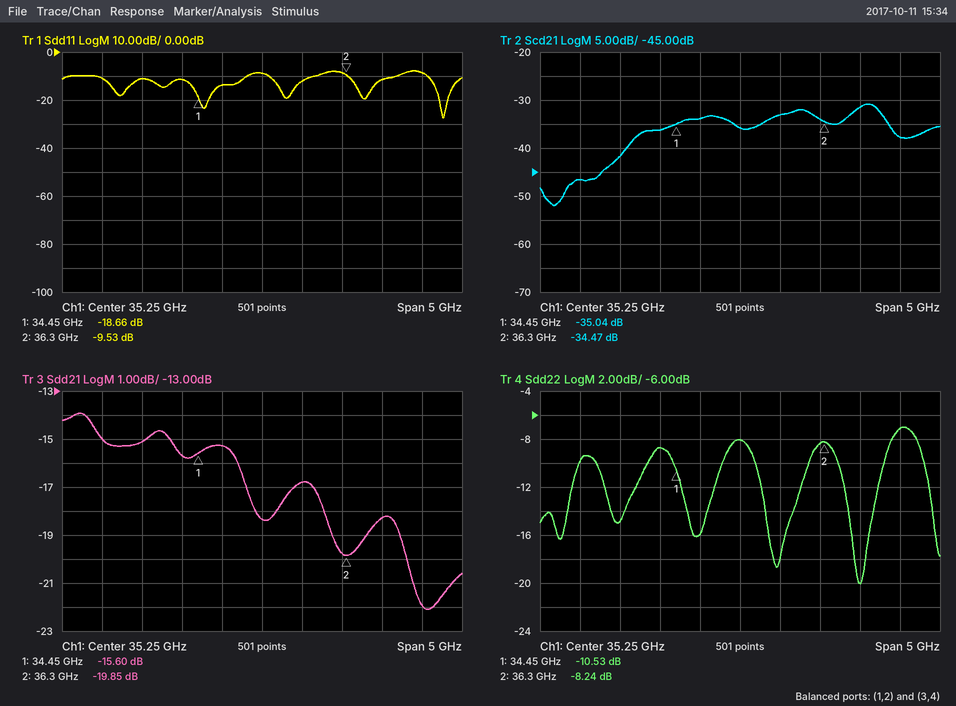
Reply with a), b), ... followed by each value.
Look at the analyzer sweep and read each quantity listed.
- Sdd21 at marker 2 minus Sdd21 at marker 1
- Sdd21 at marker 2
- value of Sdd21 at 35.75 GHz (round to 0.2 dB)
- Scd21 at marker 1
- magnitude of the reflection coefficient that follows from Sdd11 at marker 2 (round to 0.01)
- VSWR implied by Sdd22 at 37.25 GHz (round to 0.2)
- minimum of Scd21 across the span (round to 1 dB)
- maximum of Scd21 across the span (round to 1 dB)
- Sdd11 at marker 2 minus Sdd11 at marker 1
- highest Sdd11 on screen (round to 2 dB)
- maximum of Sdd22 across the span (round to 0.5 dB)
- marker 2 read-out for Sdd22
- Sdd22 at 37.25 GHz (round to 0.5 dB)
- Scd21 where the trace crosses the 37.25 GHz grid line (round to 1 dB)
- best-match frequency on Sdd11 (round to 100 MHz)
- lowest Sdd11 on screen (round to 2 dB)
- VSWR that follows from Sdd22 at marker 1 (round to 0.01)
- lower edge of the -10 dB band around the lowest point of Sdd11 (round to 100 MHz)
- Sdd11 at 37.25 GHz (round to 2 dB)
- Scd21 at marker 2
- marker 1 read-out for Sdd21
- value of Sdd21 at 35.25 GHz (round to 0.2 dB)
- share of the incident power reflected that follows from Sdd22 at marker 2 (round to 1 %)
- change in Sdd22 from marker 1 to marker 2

a) -4.25 dB
b) -19.85 dB
c) -16.8 dB
d) -35.04 dB
e) 0.33
f) 2.6
g) -52 dB
h) -31 dB
i) 9.13 dB
j) -8 dB
k) -7.0 dB
l) -8.24 dB
m) -7.0 dB
n) -38 dB
o) 37.5 GHz
p) -28 dB
q) 1.85
r) 37.3 GHz
s) -8 dB
t) -34.47 dB
u) -15.60 dB
v) -18.4 dB
w) 15 %
x) 2.29 dB
